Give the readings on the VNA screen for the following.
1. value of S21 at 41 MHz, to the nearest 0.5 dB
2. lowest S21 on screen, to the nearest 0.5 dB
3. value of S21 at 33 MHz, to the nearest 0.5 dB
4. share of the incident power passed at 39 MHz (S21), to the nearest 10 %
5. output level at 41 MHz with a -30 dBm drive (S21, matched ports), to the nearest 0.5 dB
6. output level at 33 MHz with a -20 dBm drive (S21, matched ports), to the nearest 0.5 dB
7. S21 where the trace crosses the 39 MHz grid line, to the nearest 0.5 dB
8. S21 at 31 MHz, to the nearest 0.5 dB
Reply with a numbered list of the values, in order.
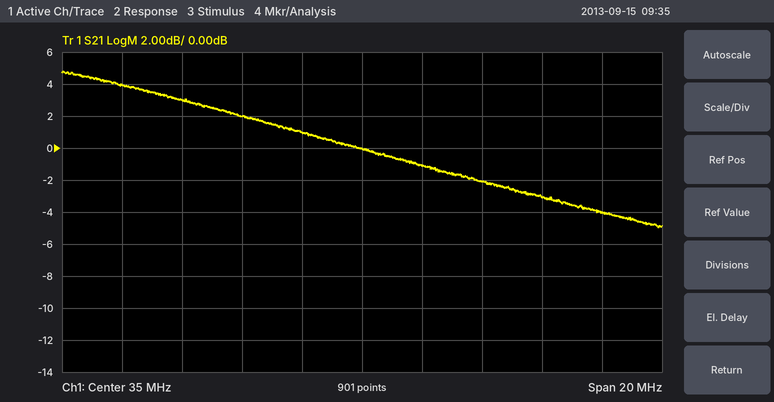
1. -3.0 dB
2. -5.0 dB
3. 1.0 dB
4. 60 %
5. -33.0 dBm
6. -19.0 dBm
7. -2.0 dB
8. 2.0 dB
